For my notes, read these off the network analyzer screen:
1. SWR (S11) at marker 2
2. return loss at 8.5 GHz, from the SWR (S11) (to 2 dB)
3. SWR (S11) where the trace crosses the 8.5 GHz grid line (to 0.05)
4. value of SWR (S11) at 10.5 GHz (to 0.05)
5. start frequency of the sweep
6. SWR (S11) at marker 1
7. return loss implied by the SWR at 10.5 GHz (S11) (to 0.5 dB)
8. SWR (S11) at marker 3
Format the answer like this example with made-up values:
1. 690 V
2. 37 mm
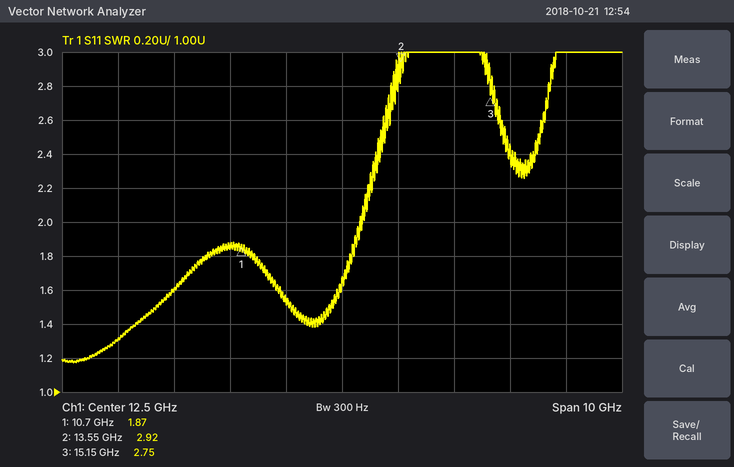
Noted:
1. 2.92
2. 18 dB
3. 1.30
4. 1.85
5. 7.5 GHz
6. 1.87
7. 10.5 dB
8. 2.75
